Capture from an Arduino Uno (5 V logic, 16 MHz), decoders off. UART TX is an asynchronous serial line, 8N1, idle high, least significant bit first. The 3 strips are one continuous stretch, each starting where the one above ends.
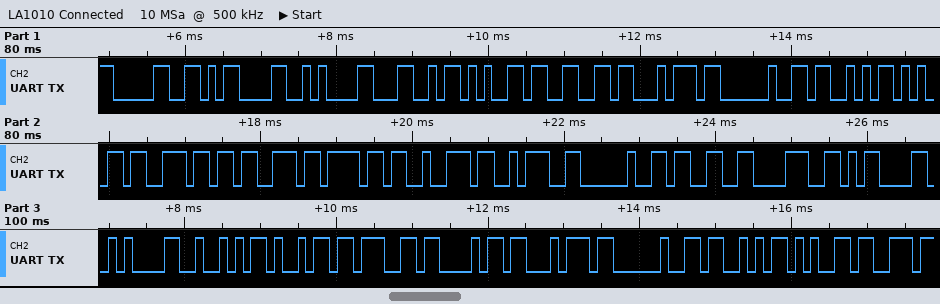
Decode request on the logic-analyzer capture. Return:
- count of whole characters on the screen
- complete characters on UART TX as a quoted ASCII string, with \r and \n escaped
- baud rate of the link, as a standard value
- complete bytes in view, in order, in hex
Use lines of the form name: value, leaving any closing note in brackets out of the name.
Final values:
count of whole characters on the screen: 28
complete characters on UART TX as a quoted ASCII string, with \r and \n escaped: "0\r\nLeft Sensor: 38\r\nRight Se"
baud rate of the link, as a standard value: 9600 baud
complete bytes in view, in order, in hex: 0x30 0x0D 0x0A 0x4C 0x65 0x66 0x74 0x20 0x53 0x65 0x6E 0x73 0x6F 0x72 0x3A 0x20 0x33 0x38 0x0D 0x0A 0x52 0x69 0x67 0x68 0x74 0x20 0x53 0x65
